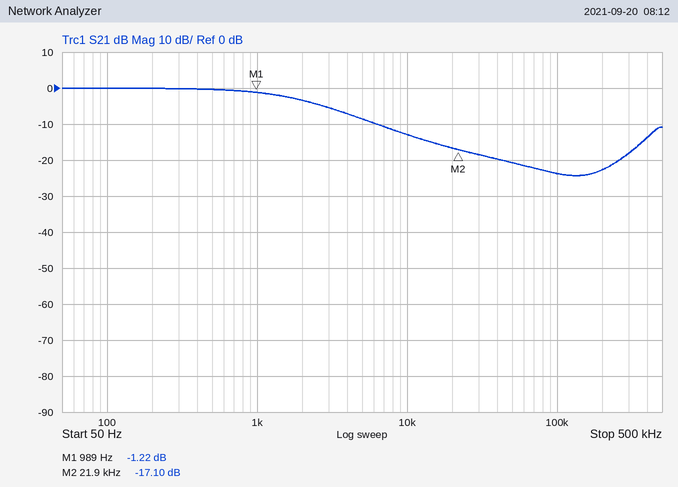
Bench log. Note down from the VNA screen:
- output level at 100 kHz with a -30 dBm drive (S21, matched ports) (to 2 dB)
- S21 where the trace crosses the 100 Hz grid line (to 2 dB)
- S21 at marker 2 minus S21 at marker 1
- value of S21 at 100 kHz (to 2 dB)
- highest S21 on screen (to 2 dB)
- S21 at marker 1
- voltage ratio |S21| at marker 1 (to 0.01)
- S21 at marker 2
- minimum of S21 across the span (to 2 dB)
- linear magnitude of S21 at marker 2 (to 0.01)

-54 dBm
0 dB
-15.88 dB
-24 dB
0 dB
-1.22 dB
0.87
-17.10 dB
-24 dB
0.14
